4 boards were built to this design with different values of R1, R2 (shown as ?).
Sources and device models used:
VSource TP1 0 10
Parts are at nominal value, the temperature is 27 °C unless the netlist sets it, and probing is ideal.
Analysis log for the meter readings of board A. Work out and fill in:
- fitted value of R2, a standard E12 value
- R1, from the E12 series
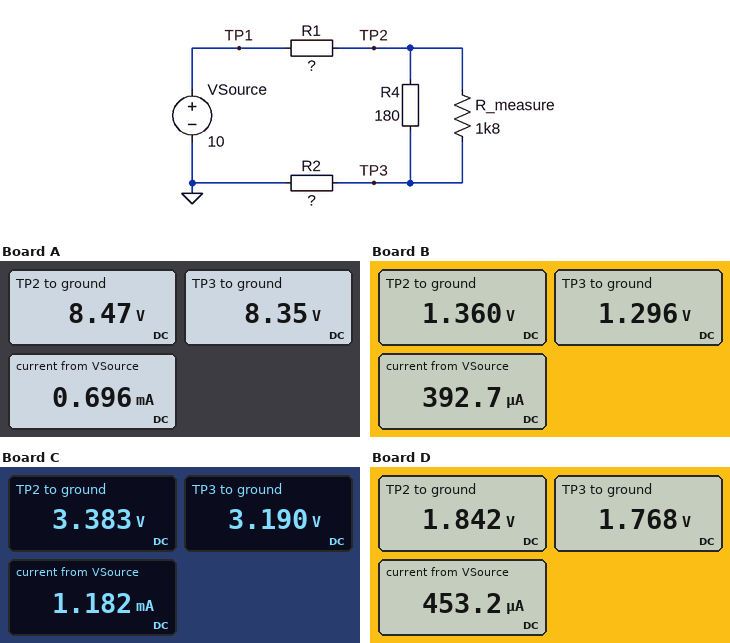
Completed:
12 kΩ
2.2 kΩ
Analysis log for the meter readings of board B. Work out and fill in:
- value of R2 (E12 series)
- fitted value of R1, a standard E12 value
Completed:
3.3 kΩ
22 kΩ
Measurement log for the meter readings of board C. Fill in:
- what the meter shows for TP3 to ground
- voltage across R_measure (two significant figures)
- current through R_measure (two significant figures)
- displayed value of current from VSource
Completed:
3.190 V
190 mV
110 µA
1.182 mA
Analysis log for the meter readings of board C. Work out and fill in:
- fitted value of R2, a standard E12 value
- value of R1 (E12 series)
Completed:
2.7 kΩ
5.6 kΩ
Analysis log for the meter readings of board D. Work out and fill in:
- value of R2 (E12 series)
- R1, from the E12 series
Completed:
3.9 kΩ
18 kΩ
